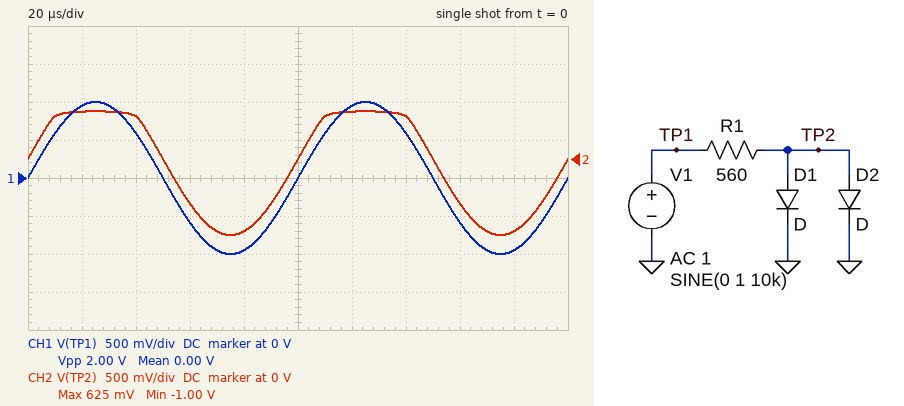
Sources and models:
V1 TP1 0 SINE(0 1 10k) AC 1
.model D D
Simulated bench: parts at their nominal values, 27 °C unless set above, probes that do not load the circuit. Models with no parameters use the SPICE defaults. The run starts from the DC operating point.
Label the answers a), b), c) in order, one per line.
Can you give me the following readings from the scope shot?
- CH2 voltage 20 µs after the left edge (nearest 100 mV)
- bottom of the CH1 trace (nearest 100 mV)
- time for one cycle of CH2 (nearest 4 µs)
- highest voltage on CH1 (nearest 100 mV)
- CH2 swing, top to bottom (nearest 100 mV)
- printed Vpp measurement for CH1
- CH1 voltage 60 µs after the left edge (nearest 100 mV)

a) 600 mV
b) -1.0 V
c) 100 µs
d) 1.0 V
e) 1.6 V
f) 2.00 V
g) -600 mV
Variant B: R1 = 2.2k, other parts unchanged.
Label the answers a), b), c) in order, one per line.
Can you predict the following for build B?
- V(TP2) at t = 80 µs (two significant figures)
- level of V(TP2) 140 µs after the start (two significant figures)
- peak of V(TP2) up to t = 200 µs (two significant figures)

a) -950 mV
b) 540 mV
c) 590 mV
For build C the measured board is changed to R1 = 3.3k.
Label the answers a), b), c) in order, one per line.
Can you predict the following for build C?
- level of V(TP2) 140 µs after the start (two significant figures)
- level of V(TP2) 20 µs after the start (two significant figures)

a) 530 mV
b) 580 mV
